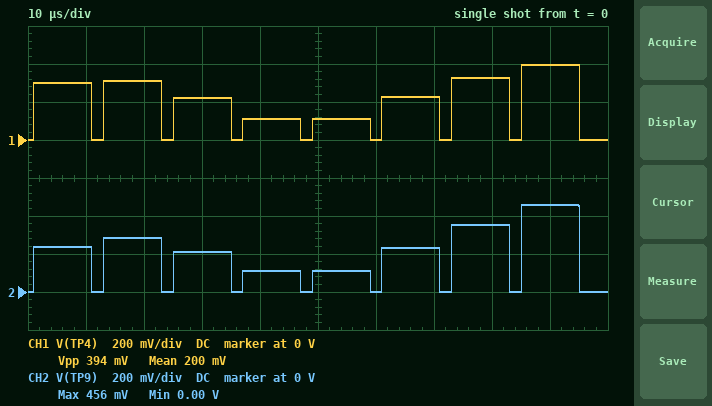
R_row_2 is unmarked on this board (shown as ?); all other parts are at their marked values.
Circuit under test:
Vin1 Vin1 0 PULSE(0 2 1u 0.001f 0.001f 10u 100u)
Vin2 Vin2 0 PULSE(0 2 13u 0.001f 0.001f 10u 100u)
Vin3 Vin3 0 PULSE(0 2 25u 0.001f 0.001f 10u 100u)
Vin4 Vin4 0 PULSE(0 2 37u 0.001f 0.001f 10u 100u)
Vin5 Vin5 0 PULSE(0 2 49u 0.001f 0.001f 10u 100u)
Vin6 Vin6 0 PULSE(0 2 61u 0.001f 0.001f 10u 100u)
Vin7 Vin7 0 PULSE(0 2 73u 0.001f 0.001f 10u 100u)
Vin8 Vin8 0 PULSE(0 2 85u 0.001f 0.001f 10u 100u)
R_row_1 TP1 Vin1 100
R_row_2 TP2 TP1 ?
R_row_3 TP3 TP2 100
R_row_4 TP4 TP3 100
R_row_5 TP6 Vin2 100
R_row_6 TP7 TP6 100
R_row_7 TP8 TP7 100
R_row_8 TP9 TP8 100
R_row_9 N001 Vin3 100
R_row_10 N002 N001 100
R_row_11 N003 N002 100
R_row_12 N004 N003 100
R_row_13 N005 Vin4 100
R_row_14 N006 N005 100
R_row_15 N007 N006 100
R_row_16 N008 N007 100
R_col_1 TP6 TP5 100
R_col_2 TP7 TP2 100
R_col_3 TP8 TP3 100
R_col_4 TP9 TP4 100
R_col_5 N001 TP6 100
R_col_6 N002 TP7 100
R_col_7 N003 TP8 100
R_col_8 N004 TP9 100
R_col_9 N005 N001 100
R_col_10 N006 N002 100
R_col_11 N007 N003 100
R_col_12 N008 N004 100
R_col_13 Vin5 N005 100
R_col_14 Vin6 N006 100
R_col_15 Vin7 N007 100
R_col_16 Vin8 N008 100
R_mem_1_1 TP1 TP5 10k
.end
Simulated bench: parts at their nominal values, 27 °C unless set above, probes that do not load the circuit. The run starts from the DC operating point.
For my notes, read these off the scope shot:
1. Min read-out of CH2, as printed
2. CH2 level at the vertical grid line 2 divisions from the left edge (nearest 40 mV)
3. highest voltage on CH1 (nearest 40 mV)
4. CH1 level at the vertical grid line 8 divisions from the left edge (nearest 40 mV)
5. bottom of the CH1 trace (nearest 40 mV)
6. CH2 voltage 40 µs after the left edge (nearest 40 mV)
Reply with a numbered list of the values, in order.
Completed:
1. 0.00 V
2. 280 mV
3. 400 mV
4. 320 mV
5. 0 V
6. 120 mV
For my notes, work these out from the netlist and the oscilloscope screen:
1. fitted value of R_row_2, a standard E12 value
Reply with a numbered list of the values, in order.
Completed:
1. 220 Ω
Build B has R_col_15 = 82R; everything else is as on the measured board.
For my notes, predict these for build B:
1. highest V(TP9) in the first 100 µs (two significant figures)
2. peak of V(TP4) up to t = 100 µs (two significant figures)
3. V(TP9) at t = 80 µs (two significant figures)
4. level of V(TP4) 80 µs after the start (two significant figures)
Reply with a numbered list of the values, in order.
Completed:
1. 440 mV
2. 380 mV
3. 400 mV
4. 370 mV
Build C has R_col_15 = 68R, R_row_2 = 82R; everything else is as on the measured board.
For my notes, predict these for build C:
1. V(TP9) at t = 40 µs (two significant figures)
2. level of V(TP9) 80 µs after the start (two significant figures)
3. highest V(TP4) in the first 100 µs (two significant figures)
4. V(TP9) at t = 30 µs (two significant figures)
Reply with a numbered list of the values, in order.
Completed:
1. 96 mV
2. 420 mV
3. 430 mV
4. 190 mV
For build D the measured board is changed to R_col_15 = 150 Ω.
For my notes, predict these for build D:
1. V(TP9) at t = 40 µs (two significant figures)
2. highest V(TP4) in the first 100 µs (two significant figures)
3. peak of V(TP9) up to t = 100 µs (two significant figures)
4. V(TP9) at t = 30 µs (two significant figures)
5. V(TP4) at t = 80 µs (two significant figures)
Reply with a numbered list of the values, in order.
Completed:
1. 120 mV
2. 420 mV
3. 480 mV
4. 220 mV
5. 250 mV
